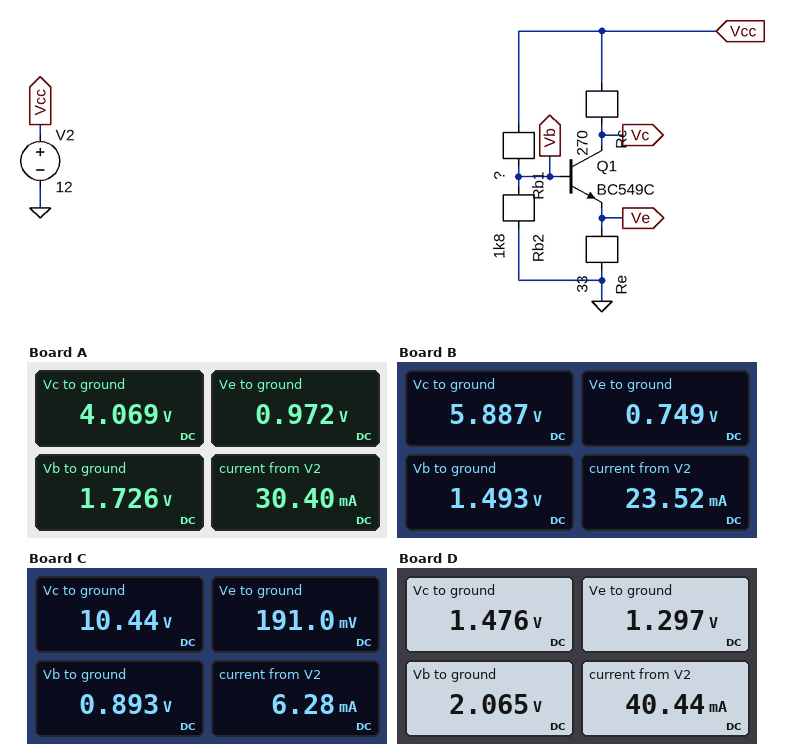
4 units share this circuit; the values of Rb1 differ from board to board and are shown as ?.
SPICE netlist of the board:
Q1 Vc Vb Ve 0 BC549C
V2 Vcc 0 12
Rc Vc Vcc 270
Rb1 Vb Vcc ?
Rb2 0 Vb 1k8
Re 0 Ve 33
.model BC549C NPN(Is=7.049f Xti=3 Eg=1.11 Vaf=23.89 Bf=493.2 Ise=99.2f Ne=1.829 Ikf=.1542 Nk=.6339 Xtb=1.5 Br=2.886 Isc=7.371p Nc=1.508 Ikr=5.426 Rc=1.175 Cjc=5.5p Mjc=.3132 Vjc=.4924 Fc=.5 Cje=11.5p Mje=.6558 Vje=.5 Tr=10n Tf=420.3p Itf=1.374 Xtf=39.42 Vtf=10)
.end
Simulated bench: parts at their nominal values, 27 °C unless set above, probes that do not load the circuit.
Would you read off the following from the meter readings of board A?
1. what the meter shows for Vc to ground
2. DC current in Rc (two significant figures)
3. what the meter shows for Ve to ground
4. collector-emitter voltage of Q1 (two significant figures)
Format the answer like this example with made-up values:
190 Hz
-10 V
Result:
4.069 V
29 mA
0.972 V
3.1 V
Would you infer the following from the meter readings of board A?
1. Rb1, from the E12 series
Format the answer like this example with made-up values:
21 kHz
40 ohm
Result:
10 kΩ
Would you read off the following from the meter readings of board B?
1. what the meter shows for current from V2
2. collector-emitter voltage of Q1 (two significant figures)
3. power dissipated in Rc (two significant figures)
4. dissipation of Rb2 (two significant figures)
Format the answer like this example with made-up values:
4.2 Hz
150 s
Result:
23.52 mA
5.1 V
140 mW
1.2 mW
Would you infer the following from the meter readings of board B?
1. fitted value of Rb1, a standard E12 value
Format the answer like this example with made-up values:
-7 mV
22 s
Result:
12 kΩ
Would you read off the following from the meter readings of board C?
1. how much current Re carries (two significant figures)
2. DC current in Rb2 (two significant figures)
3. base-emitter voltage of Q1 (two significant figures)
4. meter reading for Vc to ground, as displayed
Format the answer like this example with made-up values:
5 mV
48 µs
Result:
5.8 mA
500 µA
700 mV
10.44 V
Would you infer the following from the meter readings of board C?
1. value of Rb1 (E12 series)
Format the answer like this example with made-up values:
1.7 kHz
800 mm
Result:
22 kΩ
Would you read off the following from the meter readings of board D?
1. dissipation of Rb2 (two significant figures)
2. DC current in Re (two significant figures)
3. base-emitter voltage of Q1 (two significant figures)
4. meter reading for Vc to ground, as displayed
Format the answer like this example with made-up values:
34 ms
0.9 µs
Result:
2.4 mW
39 mA
770 mV
1.476 V
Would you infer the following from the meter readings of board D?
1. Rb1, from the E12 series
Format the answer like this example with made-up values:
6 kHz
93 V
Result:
6.8 kΩ
